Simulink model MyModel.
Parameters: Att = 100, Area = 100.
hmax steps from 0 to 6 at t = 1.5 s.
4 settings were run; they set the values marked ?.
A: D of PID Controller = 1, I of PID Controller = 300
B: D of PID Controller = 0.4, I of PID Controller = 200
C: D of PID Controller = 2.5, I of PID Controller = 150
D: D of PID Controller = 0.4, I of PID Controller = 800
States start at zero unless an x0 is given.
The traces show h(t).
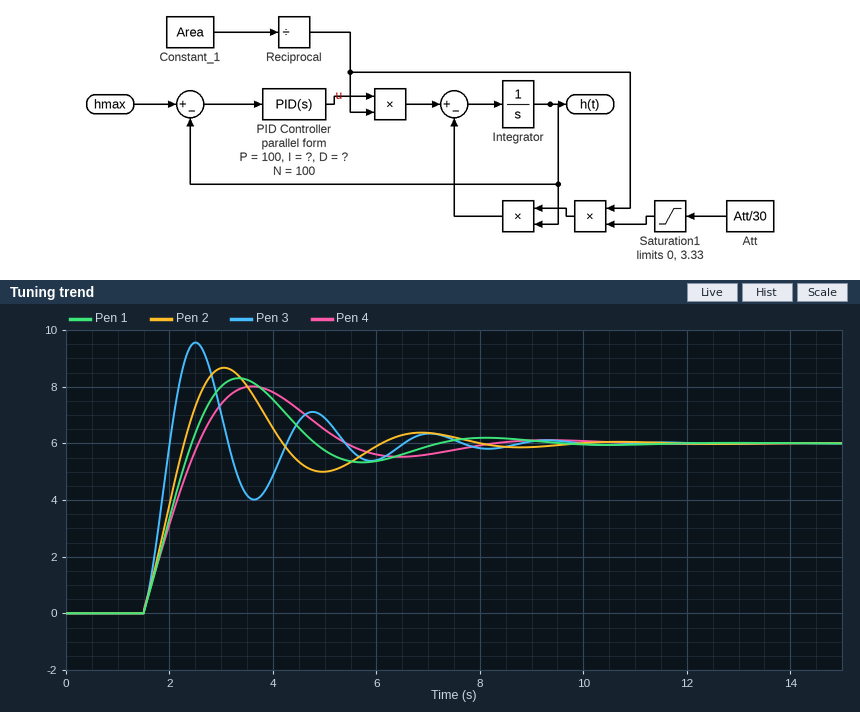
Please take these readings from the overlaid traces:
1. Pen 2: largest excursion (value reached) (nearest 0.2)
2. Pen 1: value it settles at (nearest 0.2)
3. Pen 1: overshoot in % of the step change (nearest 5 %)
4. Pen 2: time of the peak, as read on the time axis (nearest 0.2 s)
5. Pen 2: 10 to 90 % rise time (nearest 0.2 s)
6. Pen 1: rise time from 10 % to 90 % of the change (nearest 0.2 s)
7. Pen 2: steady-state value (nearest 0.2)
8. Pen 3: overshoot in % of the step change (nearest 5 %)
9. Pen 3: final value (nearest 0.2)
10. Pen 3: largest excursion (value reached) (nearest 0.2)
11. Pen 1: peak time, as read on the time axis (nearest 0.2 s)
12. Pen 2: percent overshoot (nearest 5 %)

8.6
6.0
40 %
3.0 s
0.6 s
0.8 s
6.0
60 %
6.0
9.6
3.4 s
45 %
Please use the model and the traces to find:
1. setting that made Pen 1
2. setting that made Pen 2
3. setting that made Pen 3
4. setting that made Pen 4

B
A
D
C
